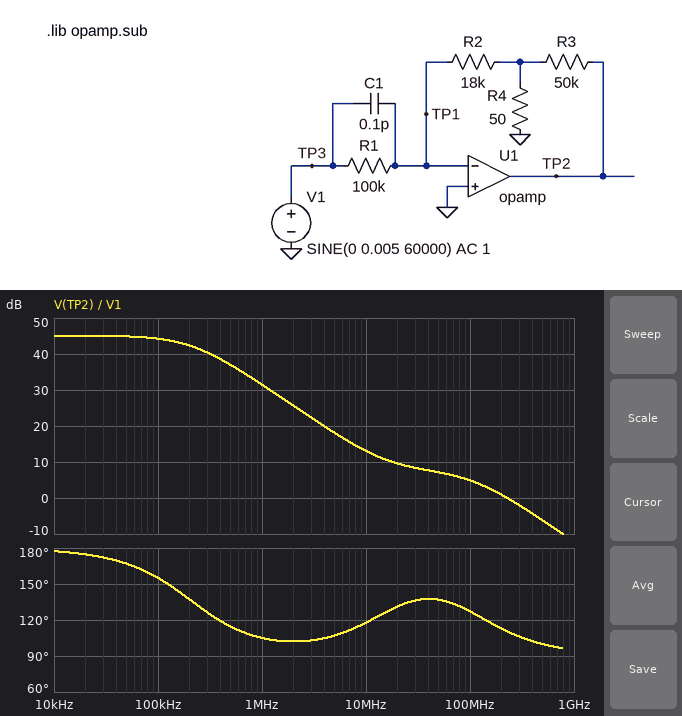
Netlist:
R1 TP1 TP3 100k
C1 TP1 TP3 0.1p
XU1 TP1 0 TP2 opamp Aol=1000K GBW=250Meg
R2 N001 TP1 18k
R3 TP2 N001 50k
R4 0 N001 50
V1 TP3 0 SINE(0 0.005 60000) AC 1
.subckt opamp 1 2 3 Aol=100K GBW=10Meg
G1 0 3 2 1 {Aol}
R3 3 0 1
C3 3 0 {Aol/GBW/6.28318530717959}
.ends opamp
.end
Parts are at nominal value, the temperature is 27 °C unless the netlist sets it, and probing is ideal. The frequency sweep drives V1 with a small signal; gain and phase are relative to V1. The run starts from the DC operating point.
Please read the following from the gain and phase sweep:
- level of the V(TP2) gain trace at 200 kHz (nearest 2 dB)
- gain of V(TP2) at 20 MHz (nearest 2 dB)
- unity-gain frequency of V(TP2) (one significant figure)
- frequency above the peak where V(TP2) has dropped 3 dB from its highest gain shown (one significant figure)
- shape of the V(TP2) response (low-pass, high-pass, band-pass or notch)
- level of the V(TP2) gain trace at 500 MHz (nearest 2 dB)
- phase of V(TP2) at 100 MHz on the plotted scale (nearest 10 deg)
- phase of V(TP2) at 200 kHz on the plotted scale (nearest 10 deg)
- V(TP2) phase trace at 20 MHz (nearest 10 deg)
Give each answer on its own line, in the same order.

42 dB
10 dB
200 MHz
200 kHz
low-pass
-6 dB
130 deg
140 deg
130 deg
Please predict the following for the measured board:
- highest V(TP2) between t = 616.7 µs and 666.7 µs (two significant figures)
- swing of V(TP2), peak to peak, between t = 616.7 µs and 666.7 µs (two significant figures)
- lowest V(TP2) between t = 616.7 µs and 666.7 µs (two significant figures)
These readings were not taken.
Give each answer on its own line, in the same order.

870 mV
1.7 V
-870 mV
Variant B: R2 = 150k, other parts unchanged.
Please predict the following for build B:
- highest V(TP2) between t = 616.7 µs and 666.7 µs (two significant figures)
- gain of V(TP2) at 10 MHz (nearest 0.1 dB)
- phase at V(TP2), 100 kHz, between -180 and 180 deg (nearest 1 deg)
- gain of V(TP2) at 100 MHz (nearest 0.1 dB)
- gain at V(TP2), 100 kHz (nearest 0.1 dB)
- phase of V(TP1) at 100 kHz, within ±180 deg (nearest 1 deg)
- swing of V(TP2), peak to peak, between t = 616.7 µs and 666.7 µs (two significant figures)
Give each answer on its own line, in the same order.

6.4 V
24.4 dB
135 deg
7.8 dB
60.5 dB
45 deg
13 V
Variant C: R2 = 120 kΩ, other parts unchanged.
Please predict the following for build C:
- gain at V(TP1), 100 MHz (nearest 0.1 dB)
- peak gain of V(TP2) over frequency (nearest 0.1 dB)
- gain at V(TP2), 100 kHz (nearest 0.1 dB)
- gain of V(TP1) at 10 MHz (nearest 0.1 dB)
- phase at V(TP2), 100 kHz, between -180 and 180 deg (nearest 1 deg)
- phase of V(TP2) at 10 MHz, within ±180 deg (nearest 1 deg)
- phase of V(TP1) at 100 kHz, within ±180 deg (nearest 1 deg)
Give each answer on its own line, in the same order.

-0.2 dB
61.6 dB
59.1 dB
-4.3 dB
139 deg
104 deg
49 deg
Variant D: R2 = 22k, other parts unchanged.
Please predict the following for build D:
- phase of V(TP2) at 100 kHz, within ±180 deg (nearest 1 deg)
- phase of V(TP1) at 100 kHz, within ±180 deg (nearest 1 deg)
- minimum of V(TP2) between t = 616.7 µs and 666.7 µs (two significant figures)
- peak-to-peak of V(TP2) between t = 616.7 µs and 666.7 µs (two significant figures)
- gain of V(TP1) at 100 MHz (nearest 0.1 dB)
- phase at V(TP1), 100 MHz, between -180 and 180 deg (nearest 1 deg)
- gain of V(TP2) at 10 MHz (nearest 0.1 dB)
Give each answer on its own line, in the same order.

154 deg
64 deg
-1.1 V
2.1 V
-2.4 dB
32 deg
14.5 dB
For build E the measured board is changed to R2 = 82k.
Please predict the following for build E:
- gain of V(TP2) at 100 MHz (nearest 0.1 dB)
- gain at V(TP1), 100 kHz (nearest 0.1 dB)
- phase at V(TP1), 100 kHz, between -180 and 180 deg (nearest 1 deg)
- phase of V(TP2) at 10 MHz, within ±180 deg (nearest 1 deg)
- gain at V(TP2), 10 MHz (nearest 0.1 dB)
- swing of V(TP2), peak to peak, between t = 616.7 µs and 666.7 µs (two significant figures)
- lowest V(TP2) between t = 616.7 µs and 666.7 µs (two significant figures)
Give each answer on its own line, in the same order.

7.6 dB
-11.5 dB
54 deg
107 deg
22.2 dB
7.5 V
-3.8 V
